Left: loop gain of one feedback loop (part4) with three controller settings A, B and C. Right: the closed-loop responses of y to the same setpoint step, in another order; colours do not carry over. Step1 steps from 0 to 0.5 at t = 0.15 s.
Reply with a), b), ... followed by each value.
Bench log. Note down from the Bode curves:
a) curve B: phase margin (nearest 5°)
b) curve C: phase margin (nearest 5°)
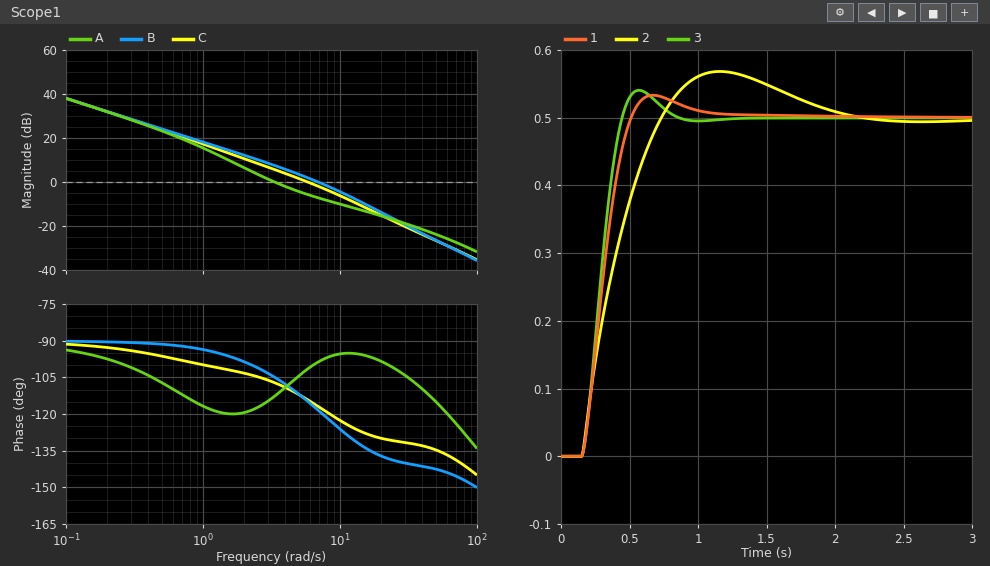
a) 60°
b) 65°
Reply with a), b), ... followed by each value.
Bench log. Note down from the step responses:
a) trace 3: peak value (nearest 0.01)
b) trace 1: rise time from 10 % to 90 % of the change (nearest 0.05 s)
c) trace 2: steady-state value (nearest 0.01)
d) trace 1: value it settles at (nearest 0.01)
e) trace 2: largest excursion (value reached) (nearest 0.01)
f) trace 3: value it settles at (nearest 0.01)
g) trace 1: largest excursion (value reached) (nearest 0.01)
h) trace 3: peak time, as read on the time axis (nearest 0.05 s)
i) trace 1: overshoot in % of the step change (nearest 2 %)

a) 0.54
b) 0.25 s
c) 0.50
d) 0.50
e) 0.57
f) 0.50
g) 0.53
h) 0.55 s
i) 6 %
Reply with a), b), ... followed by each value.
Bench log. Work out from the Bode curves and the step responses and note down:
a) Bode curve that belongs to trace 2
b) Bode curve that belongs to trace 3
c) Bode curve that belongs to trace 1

a) A
b) B
c) C
